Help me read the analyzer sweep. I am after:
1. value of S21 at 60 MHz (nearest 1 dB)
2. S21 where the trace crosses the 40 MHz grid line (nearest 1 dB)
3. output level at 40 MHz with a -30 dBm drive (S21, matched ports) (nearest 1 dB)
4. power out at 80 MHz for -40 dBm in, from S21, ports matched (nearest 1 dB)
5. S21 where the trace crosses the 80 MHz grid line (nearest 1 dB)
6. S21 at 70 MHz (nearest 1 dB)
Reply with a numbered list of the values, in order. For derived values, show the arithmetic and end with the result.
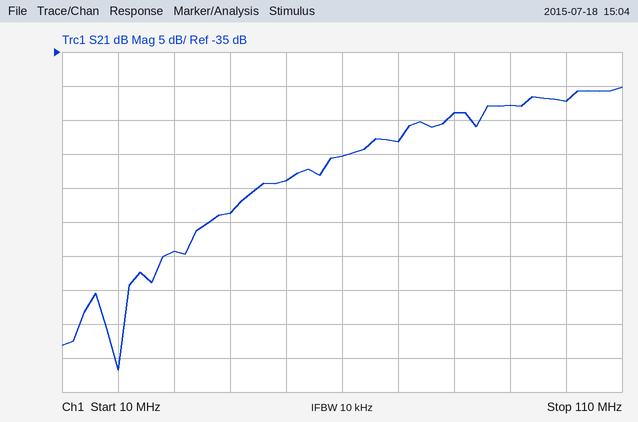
1. -50 dB
2. -59 dB
3. -30 dBm + (-59 dB) = -89 dBm
4. -40 dBm + (-44 dB) = -84 dBm
5. -44 dB
6. -48 dB
